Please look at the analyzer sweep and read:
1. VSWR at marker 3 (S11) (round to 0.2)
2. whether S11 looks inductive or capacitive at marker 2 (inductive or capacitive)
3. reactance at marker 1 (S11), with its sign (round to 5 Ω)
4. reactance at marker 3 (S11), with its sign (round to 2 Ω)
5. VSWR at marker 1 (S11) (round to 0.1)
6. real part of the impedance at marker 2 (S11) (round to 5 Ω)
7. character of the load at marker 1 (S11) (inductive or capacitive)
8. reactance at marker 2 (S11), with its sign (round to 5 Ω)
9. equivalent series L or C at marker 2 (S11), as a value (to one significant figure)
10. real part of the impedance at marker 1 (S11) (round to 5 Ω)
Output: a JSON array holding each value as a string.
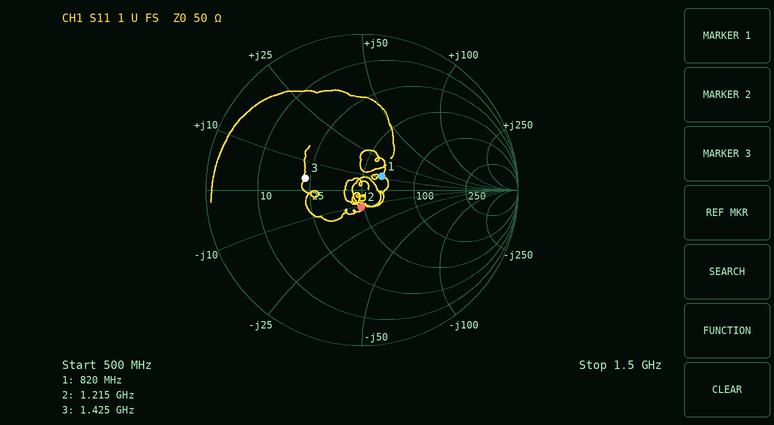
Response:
["2.2", "capacitive", "+10 Ω", "+4 Ω", "1.4", "50 Ω", "inductive", "-10 Ω", "10 pF", "65 Ω"]
